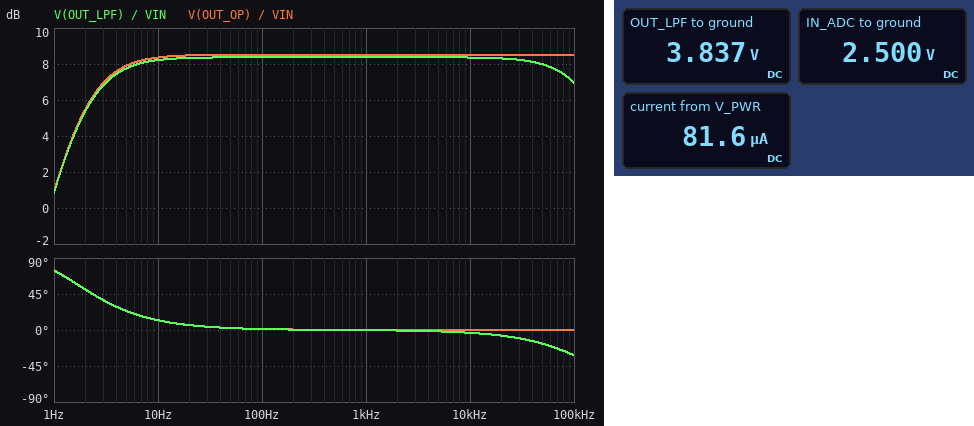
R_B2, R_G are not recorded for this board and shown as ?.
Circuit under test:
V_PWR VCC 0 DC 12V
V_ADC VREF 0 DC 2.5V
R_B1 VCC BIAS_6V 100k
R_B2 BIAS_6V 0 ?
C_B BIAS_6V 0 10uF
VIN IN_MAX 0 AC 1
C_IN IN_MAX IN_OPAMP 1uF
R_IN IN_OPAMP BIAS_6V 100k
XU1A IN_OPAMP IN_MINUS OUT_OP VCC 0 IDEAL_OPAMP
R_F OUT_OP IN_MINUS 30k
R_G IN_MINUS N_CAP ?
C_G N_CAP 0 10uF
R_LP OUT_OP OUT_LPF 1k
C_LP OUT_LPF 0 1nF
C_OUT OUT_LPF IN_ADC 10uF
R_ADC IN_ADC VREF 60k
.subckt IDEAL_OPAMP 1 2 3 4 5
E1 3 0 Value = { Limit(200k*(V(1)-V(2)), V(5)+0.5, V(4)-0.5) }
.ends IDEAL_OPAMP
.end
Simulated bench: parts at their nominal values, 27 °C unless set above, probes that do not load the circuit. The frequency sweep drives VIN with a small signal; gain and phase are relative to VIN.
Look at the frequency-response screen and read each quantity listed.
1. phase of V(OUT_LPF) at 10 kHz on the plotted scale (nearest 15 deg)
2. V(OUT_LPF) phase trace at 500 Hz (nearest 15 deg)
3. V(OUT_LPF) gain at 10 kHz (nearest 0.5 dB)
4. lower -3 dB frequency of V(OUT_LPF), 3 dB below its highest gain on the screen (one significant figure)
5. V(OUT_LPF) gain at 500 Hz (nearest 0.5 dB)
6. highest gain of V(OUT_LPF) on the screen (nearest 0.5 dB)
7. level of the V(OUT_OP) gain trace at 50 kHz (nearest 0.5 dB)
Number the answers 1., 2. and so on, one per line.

1. 0 deg
2. 0 deg
3. 8.5 dB
4. 2 Hz
5. 8.5 dB
6. 8.5 dB
7. 8.5 dB
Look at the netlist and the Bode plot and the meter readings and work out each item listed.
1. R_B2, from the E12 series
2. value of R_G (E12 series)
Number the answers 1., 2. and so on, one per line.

1. 47 kΩ
2. 18 kΩ
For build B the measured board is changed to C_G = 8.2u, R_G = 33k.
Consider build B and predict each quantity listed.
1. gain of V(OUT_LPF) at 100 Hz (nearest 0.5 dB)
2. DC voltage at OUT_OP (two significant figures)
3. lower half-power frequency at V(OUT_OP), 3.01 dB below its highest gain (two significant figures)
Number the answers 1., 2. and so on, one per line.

1. 5.5 dB
2. 3.8 V
3. 1.8 Hz
